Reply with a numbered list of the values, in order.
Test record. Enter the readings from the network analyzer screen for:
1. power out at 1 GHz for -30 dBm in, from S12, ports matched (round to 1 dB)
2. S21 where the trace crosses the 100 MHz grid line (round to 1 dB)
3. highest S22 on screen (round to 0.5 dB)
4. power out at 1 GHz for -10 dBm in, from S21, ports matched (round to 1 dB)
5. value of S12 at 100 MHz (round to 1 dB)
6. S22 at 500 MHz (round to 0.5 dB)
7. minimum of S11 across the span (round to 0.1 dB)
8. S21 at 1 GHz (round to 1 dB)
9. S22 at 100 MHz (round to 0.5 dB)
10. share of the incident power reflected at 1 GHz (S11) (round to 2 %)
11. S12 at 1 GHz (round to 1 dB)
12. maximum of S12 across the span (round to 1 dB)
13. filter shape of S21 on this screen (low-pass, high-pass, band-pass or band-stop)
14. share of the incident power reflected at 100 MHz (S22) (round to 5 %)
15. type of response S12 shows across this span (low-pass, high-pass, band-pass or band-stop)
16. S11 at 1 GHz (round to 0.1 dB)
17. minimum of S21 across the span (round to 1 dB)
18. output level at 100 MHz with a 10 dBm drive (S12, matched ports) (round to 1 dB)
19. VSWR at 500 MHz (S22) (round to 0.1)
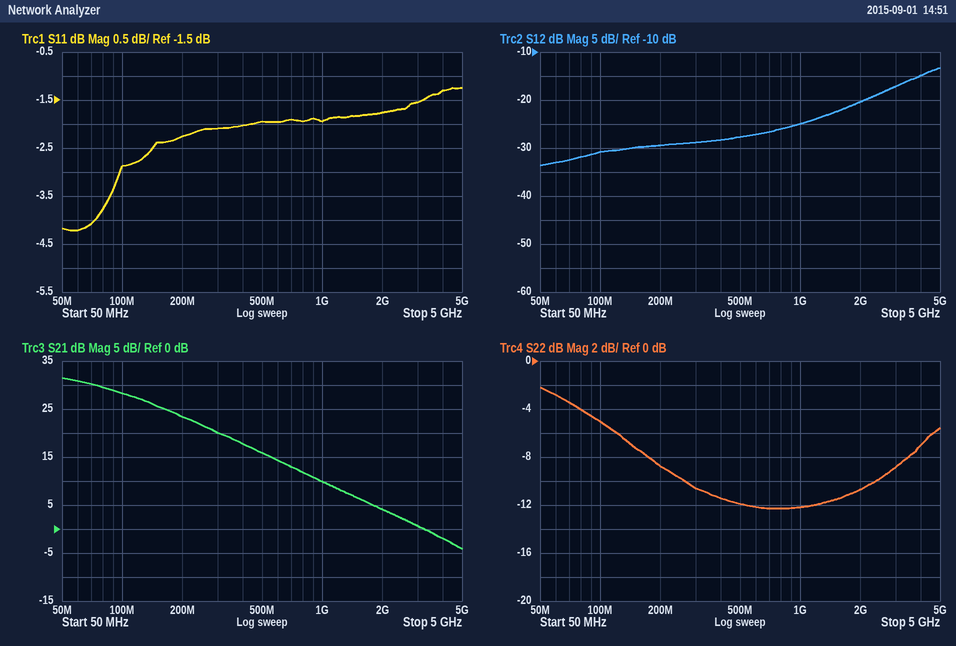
1. -55 dBm
2. 28 dB
3. -2.0 dB
4. 0 dBm
5. -31 dB
6. -12.0 dB
7. -4.2 dB
8. 10 dB
9. -5.0 dB
10. 64 %
11. -25 dB
12. -13 dB
13. low-pass
14. 30 %
15. high-pass
16. -1.9 dB
17. -4 dB
18. -21 dBm
19. 1.7
